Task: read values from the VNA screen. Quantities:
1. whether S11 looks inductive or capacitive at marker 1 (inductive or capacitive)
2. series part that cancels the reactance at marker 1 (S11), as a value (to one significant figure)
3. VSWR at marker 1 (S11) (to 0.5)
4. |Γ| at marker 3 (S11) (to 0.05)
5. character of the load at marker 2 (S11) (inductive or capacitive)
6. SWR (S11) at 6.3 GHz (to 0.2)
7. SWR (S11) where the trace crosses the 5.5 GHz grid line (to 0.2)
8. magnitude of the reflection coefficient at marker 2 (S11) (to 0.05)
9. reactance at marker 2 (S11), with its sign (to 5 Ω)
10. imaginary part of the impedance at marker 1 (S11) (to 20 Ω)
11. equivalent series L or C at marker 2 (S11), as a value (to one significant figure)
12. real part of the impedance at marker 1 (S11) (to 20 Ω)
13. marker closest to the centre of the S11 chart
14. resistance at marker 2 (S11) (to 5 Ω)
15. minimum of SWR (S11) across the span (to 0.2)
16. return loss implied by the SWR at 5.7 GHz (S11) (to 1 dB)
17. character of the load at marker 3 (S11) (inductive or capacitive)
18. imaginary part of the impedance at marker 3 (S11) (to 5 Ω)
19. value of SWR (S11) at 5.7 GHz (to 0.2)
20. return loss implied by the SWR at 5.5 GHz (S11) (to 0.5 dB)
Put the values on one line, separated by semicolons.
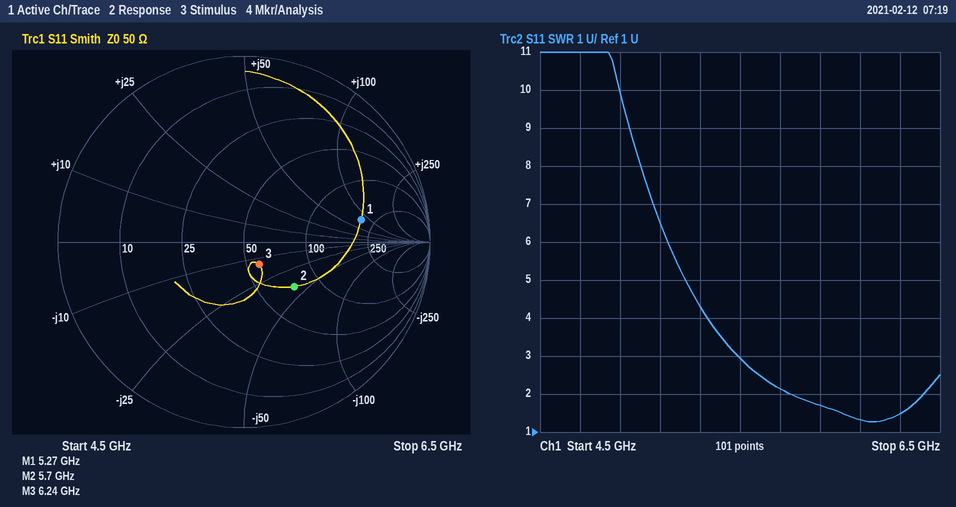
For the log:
inductive; 400 fF; 4.5; 0.15; capacitive; 1.4; 3.0; 0.35; -40 Ω; +80 Ω; 700 fF; 200 Ω; marker 3; 75 Ω; 1.2; 9 dB; capacitive; -15 Ω; 2.2; 6.0 dB
